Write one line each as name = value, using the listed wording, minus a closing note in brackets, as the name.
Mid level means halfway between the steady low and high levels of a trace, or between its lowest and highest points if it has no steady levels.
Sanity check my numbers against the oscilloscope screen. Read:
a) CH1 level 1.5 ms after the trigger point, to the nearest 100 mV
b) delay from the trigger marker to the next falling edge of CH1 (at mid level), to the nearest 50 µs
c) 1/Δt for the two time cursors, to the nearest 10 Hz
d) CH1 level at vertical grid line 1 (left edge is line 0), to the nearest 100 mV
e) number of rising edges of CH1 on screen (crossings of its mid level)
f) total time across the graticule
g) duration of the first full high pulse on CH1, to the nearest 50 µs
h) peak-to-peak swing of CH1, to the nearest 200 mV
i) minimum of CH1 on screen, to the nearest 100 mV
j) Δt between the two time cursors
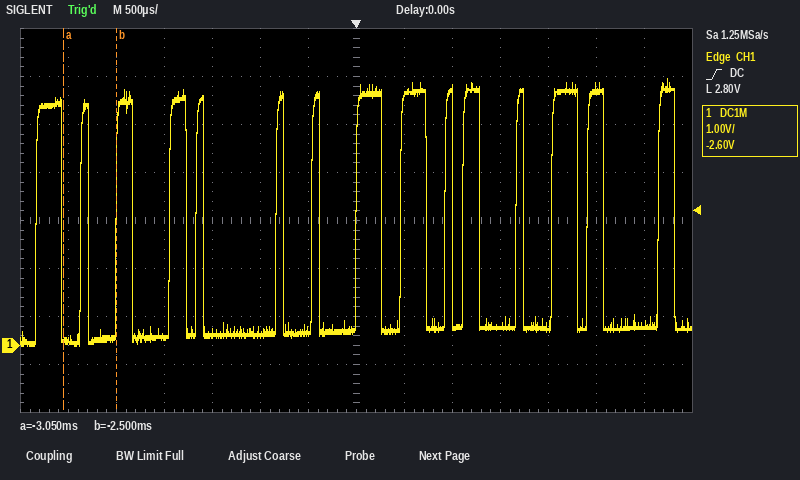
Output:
CH1 level 1.5 ms after the trigger point, to the nearest 100 mV = 400 mV
delay from the trigger marker to the next falling edge of CH1 (at mid level), to the nearest 50 µs = 250 µs
1/Δt for the two time cursors, to the nearest 10 Hz = 1.82 kHz
CH1 level at vertical grid line 1 (left edge is line 0), to the nearest 100 mV = 100 mV
number of rising edges of CH1 on screen = 15
total time across the graticule = 7 ms
duration of the first full high pulse on CH1, to the nearest 50 µs = 250 µs
peak-to-peak swing of CH1, to the nearest 200 mV = 5.6 V
minimum of CH1 on screen, to the nearest 100 mV = 0.0 V
Δt between the two time cursors = 550 µs
